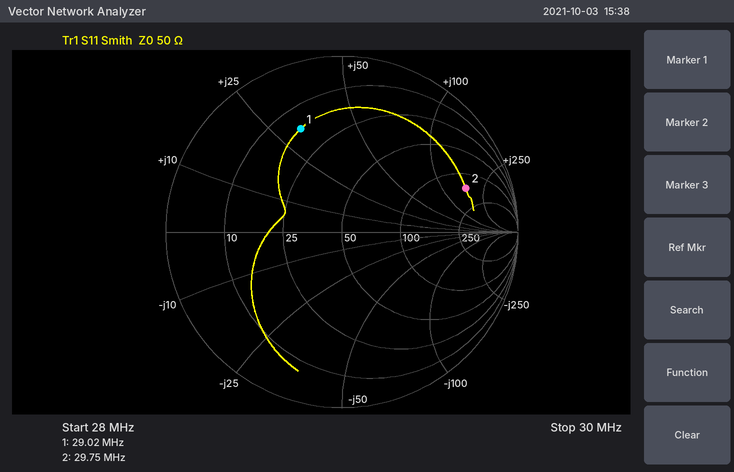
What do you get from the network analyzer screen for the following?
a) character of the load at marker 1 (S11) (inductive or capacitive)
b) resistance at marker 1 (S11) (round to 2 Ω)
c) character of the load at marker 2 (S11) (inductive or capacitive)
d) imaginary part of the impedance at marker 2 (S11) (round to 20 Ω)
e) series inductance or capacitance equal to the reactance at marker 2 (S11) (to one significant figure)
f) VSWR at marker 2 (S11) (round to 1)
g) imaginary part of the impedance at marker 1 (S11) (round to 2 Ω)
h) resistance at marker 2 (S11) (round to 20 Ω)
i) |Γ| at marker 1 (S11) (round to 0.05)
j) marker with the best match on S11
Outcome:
inductive
16 Ω
inductive
+160 Ω
900 nH
7
+32 Ω
140 Ω
0.65
marker 1
